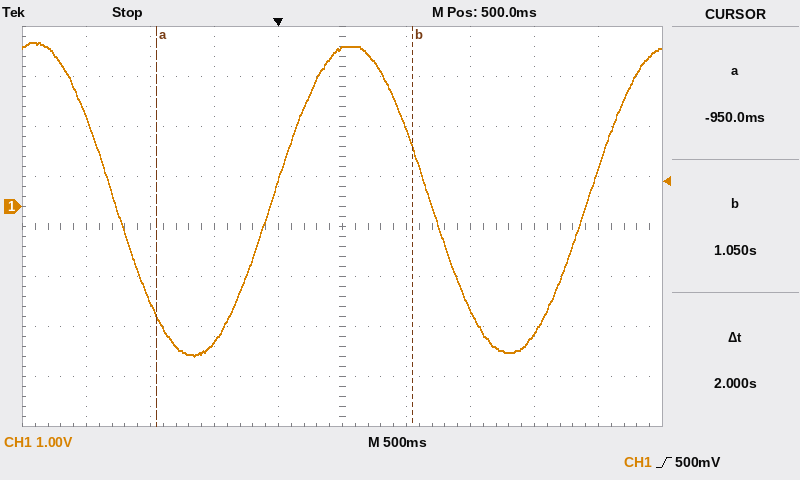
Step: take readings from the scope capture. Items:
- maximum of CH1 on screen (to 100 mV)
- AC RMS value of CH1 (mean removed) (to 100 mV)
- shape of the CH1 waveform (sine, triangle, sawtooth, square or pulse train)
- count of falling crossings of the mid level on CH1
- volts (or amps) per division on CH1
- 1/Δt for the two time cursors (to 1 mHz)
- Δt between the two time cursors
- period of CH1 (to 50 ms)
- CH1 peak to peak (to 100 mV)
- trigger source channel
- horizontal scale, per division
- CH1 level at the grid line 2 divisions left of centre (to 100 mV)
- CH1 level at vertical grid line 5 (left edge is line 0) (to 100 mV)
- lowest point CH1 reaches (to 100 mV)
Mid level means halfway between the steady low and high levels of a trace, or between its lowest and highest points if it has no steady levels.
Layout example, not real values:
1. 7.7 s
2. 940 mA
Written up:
1. 3.3 V
2. 2.2 V
3. sine
4. 2
5. 1 V
6. 500 mHz
7. 2 s
8. 2.45 s
9. 6.3 V
10. CH1
11. 500 ms
12. -2.7 V
13. 3.2 V
14. -3.0 V
